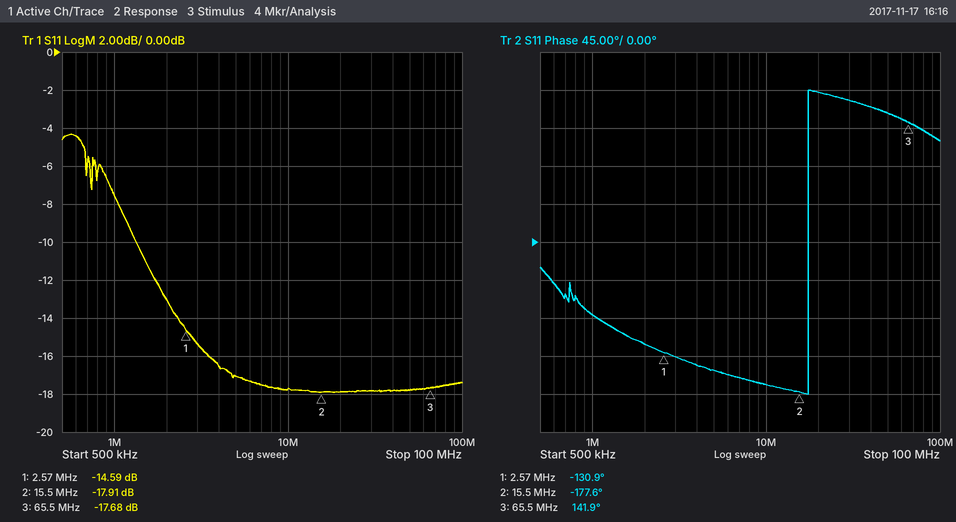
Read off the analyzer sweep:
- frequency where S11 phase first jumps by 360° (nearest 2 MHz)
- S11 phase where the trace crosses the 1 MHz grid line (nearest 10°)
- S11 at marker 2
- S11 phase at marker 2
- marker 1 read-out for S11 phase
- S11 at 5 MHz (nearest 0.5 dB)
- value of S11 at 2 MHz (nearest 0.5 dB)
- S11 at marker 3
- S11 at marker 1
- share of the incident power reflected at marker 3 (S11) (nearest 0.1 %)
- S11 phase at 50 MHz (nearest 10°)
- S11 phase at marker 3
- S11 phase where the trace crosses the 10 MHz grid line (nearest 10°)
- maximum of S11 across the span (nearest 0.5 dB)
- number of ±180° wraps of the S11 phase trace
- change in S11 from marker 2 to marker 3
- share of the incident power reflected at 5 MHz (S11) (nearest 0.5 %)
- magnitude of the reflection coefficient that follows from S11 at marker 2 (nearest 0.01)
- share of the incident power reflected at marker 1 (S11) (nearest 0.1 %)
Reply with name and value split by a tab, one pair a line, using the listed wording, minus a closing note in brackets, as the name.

frequency where S11 phase first jumps by 360°	18 MHz
S11 phase where the trace crosses the 1 MHz grid line	-90°
S11 at marker 2	-17.91 dB
S11 phase at marker 2	-177.6°
marker 1 read-out for S11 phase	-130.9°
S11 at 5 MHz	-17.0 dB
value of S11 at 2 MHz	-13.0 dB
S11 at marker 3	-17.68 dB
S11 at marker 1	-14.59 dB
share of the incident power reflected at marker 3 (S11)	1.7 %
S11 phase at 50 MHz	150°
S11 phase at marker 3	141.9°
S11 phase where the trace crosses the 10 MHz grid line	-170°
maximum of S11 across the span	-4.5 dB
number of ±180° wraps of the S11 phase trace	1
change in S11 from marker 2 to marker 3	0.23 dB
share of the incident power reflected at 5 MHz (S11)	2.0 %
magnitude of the reflection coefficient that follows from S11 at marker 2	0.13
share of the incident power reflected at marker 1 (S11)	3.5 %
